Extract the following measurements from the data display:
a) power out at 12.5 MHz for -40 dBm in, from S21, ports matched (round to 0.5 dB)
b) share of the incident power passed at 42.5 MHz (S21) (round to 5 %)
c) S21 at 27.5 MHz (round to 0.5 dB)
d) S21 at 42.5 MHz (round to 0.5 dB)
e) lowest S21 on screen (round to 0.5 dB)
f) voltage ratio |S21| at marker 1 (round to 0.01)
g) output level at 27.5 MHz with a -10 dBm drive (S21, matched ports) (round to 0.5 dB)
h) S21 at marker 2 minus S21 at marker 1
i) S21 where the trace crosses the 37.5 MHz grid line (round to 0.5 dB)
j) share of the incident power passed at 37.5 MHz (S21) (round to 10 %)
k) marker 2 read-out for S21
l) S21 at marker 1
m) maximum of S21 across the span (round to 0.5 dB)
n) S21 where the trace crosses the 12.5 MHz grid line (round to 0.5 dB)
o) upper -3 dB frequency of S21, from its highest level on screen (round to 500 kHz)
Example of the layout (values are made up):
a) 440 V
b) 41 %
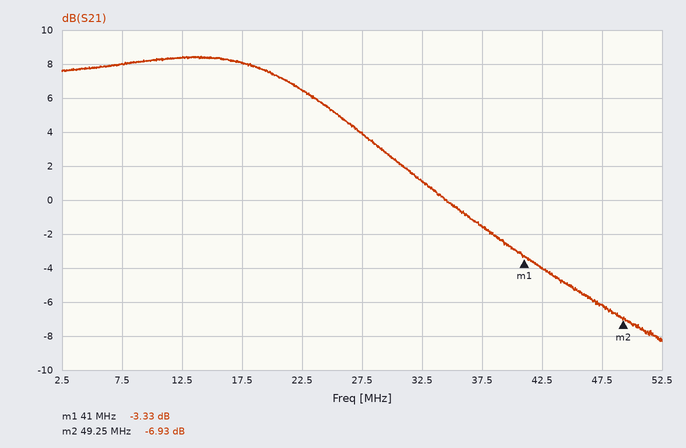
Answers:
a) -31.5 dBm
b) 40 %
c) 4.0 dB
d) -4.0 dB
e) -8.5 dB
f) 0.68
g) -6.0 dBm
h) -3.60 dB
i) -1.5 dB
j) 70 %
k) -6.93 dB
l) -3.33 dB
m) 8.5 dB
n) 8.5 dB
o) 24.5 MHz
